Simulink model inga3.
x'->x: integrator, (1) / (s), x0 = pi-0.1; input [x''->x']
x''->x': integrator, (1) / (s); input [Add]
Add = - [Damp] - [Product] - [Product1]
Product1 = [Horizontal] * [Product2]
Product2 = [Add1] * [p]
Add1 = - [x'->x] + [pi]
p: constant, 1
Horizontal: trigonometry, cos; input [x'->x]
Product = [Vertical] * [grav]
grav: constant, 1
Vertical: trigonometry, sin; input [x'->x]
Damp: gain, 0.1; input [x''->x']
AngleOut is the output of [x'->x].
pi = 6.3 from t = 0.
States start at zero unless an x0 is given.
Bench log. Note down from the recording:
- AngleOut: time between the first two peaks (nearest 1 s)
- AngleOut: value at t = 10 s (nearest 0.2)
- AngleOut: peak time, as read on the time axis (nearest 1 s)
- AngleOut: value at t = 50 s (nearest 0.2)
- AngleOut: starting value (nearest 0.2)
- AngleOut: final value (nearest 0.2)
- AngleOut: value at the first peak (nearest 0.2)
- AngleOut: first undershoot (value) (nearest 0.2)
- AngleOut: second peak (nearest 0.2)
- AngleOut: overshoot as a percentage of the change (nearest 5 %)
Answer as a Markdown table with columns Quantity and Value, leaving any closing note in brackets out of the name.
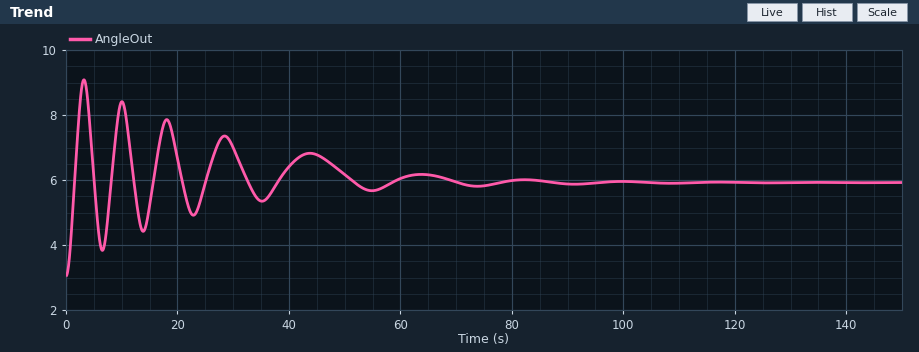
| Quantity | Value |
|---|---|
| AngleOut: time between the first two peaks | 7 s |
| AngleOut: value at t = 10 s | 8.4 |
| AngleOut: peak time, as read on the time axis | 3 s |
| AngleOut: value at t = 50 s | 6.2 |
| AngleOut: starting value | 3.0 |
| AngleOut: final value | 6.0 |
| AngleOut: value at the first peak | 9.0 |
| AngleOut: first undershoot (value) | 3.8 |
| AngleOut: second peak | 8.4 |
| AngleOut: overshoot as a percentage of the change | 110 % |
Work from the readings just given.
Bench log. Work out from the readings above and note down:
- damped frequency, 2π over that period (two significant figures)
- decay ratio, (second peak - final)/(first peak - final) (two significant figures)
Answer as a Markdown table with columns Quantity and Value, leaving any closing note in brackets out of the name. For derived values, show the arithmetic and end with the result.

| Quantity | Value |
|---|---|
| damped frequency, 2π over that period | 2π / 7 = 0.90 rad/s |
| decay ratio, (second peak - final)/(first peak - final) | (8.4 - 6) / (9 - 6) = 0.80 |
